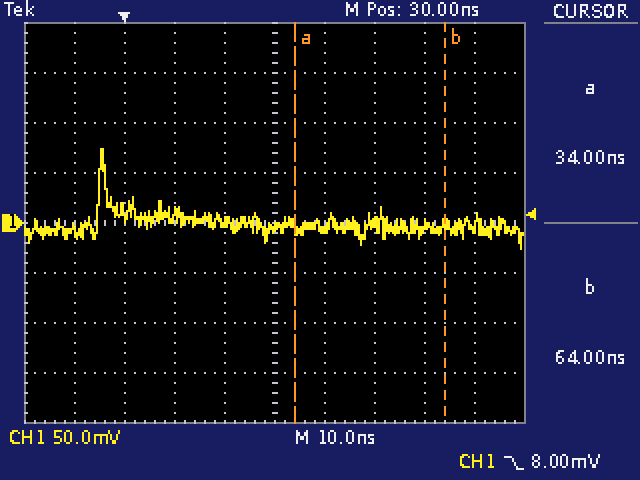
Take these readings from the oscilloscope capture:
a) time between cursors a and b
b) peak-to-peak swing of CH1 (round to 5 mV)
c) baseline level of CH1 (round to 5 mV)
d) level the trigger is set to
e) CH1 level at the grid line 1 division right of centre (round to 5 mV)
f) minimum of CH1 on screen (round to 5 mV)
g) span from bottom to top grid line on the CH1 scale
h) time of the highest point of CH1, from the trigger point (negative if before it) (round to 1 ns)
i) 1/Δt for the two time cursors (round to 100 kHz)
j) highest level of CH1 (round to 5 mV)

30 ns
100 mV
-5 mV
8.00 mV
-5 mV
-25 mV
400 mV
-4 ns
33.3 MHz
75 mV
